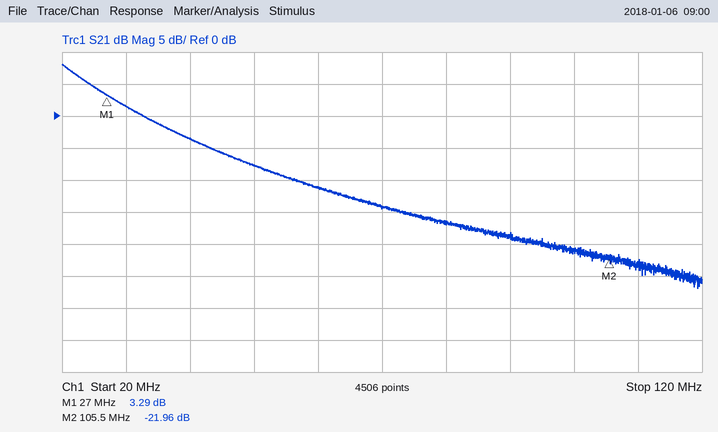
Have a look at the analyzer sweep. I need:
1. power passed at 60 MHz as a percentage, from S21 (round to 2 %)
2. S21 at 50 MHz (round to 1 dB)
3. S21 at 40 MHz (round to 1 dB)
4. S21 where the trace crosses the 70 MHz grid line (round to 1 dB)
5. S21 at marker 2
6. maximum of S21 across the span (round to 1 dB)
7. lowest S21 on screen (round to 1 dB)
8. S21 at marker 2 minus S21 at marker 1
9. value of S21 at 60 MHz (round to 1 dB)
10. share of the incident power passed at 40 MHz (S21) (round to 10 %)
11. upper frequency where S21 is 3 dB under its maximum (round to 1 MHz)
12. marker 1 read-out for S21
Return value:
8 %
-8 dB
-4 dB
-14 dB
-21.96 dB
8 dB
-27 dB
-25.25 dB
-11 dB
40 %
24 MHz
3.29 dB
